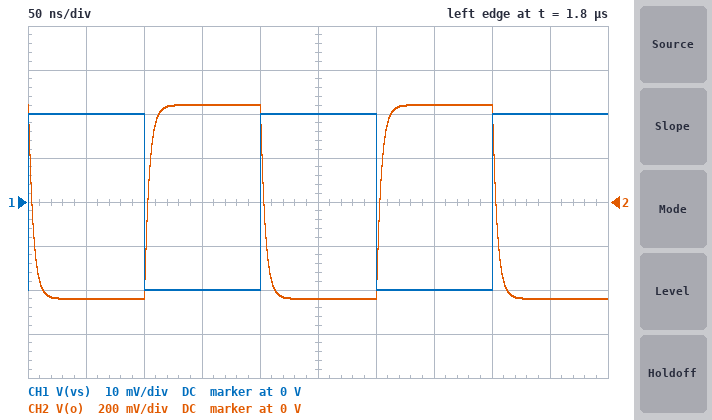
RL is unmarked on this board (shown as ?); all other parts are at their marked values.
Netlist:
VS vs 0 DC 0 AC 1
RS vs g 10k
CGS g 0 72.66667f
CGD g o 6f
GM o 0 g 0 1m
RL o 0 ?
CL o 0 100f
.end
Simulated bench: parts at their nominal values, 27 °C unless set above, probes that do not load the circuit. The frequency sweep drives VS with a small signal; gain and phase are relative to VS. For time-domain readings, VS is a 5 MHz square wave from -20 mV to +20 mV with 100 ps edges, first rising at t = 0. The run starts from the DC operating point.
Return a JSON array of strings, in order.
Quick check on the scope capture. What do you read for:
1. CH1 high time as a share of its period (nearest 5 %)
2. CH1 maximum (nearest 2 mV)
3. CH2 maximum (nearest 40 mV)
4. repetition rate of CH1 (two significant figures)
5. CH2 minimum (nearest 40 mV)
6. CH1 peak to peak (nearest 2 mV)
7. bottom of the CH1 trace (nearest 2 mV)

["50 %", "20 mV", "440 mV", "5.0 MHz", "-440 mV", "40 mV", "-20 mV"]
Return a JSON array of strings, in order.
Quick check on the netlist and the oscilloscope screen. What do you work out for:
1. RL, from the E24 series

["22 kΩ"]
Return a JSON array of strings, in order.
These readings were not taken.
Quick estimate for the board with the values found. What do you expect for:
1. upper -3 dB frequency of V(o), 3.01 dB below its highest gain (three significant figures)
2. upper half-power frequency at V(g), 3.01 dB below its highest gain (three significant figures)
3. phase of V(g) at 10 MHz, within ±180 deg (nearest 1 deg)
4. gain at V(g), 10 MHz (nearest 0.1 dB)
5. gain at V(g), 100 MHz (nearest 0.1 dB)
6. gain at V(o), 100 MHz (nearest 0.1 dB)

["39.5 MHz", "66.4 MHz", "-7 deg", "-0.2 dB", "-4.0 dB", "17.9 dB"]
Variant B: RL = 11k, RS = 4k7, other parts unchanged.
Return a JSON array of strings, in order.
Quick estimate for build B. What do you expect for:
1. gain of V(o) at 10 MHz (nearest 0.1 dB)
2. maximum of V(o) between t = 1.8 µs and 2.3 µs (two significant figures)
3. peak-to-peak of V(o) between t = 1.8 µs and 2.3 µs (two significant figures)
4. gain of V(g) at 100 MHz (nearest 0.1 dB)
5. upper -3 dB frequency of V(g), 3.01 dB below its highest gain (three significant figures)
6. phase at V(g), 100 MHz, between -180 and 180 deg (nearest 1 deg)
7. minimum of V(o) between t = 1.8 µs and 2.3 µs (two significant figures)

["20.8 dB", "220 mV", "440 mV", "-1.2 dB", "268 MHz", "-18 deg", "-220 mV"]
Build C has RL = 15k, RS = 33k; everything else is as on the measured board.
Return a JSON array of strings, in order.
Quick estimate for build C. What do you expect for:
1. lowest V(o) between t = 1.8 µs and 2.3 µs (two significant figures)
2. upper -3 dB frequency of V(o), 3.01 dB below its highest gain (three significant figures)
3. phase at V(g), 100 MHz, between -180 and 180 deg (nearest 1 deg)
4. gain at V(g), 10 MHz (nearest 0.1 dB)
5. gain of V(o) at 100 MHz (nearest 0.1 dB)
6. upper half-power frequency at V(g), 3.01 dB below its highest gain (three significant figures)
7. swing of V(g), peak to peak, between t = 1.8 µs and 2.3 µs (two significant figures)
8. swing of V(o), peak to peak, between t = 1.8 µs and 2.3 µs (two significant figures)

["-300 mV", "24.2 MHz", "-53 deg", "-0.6 dB", "10.4 dB", "25.7 MHz", "40 mV", "600 mV"]
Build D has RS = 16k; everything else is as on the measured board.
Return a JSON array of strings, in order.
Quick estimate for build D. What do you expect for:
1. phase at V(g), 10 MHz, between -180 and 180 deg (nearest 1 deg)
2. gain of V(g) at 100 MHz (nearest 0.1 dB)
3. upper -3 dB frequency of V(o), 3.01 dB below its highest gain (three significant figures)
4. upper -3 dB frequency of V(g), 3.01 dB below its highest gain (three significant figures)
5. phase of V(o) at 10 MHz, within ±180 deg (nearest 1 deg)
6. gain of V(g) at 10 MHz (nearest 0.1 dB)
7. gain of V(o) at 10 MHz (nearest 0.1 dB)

["-12 deg", "-6.1 dB", "30.6 MHz", "39.4 MHz", "160 deg", "-0.3 dB", "26.4 dB"]
